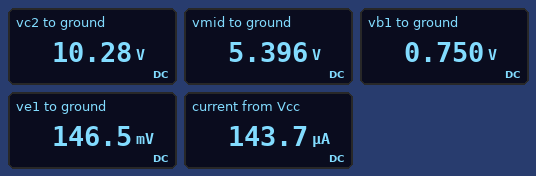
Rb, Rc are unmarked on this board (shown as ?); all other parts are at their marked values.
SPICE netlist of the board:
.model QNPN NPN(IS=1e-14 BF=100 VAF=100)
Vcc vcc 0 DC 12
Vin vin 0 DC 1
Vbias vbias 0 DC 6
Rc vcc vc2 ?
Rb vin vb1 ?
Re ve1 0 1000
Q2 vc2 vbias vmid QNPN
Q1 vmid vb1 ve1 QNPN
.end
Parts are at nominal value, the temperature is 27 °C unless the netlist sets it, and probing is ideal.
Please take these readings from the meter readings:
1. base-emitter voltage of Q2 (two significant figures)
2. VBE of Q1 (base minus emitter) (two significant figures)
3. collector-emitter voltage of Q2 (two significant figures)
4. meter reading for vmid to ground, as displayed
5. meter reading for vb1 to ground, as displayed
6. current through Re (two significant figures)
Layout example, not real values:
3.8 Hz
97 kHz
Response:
600 mV
600 mV
4.9 V
5.396 V
0.750 V
150 µA
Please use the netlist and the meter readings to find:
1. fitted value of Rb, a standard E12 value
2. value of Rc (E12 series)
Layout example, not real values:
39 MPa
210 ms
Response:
180 kΩ
12 kΩ
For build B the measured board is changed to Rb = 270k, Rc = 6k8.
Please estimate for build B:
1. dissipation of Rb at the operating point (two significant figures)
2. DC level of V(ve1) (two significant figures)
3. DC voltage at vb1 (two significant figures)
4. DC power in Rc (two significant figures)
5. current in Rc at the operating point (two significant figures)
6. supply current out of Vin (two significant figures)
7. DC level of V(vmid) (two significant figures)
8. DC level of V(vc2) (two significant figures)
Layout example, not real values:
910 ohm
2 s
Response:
310 nW
110 mV
710 mV
84 µW
110 µA
1.1 µA
5.4 V
11 V
